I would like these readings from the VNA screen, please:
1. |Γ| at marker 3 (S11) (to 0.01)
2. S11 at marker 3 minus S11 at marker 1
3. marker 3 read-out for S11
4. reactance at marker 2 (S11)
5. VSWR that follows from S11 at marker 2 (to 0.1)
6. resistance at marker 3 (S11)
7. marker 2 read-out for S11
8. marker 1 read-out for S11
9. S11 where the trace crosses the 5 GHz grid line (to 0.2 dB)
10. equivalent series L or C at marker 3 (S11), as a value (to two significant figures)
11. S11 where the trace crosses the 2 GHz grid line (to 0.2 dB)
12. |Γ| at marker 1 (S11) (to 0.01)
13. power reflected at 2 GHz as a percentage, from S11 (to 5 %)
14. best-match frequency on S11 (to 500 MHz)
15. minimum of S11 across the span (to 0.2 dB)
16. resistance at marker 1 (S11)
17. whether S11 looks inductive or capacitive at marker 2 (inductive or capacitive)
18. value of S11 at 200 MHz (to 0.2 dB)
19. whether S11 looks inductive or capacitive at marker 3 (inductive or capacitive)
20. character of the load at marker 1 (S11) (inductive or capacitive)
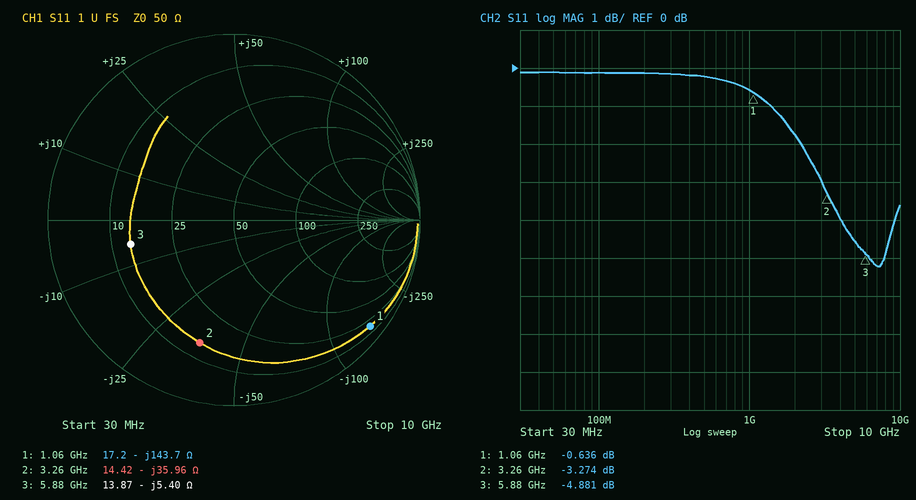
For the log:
0.57
-4.245 dB
-4.881 dB
-35.96 Ω
5.4
13.87 Ω
-3.274 dB
-0.636 dB
-4.6 dB
5.0 pF
-1.8 dB
0.93
65 %
7.0 GHz
-5.2 dB
17.2 Ω
capacitive
-0.2 dB
capacitive
capacitive
